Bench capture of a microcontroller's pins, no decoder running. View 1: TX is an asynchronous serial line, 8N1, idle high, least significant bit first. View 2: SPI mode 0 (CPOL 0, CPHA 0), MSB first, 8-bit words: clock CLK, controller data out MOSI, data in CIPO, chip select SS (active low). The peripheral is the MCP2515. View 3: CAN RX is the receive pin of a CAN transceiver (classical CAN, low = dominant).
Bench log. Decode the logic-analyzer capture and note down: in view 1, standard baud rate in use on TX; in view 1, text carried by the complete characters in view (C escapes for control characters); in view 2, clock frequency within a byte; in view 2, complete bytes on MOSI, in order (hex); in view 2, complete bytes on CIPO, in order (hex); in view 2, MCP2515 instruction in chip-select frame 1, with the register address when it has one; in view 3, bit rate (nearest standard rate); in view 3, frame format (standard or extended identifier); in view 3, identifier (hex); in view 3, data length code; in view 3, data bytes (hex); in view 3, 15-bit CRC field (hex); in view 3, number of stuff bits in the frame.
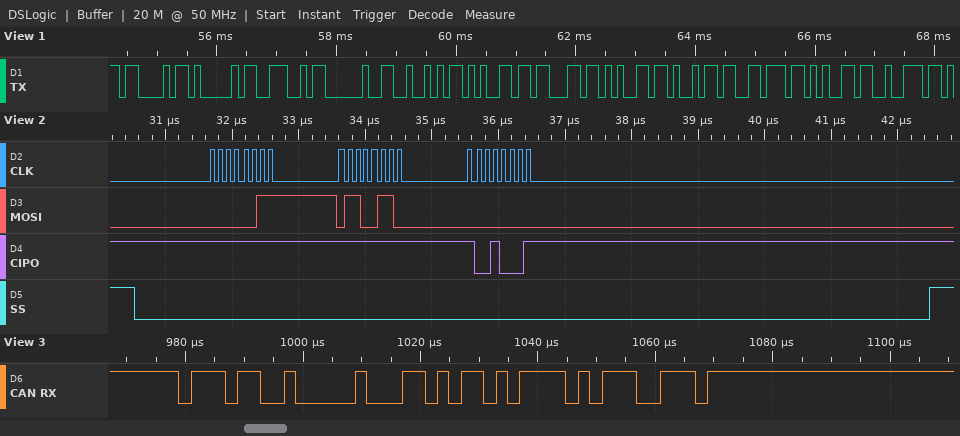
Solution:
9600 baud
"CAN Receiver"
8 MHz
03 66 00
FF FF 91
READ 0x66
500 kbit/s
standard
0x764
1
AD
0x3D73
1
